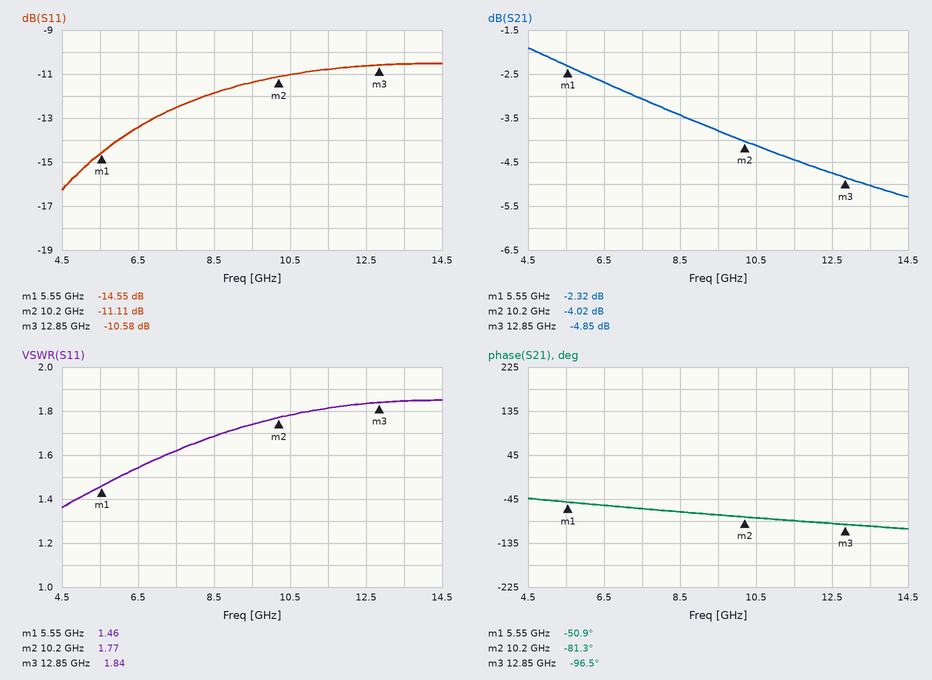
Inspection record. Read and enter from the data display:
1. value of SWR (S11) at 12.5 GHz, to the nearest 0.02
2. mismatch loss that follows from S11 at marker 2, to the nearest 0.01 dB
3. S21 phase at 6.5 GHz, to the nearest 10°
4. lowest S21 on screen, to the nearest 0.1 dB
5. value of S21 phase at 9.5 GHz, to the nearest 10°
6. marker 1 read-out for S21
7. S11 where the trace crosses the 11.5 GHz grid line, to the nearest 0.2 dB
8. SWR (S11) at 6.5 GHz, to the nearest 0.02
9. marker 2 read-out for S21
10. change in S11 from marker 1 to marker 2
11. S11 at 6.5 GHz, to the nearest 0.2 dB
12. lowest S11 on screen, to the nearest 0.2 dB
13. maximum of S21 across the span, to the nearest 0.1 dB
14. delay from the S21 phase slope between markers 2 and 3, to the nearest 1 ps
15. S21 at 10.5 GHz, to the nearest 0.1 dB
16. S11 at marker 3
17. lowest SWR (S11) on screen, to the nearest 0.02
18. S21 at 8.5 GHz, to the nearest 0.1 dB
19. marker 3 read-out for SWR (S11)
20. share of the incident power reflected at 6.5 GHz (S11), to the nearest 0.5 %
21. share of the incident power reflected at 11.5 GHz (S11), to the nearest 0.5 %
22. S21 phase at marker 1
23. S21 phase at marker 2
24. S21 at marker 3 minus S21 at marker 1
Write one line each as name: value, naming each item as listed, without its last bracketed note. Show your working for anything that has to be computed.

value of SWR (S11) at 12.5 GHz, to the nearest 0.02: 1.84
mismatch loss that follows from S11 at marker 2, to the nearest 0.01 dB: −10 log10(1 − 10^(-11.11/10)) ≈ 0.35 dB
S21 phase at 6.5 GHz, to the nearest 10°: -60°
lowest S21 on screen, to the nearest 0.1 dB: -5.3 dB
value of S21 phase at 9.5 GHz, to the nearest 10°: -80°
marker 1 read-out for S21: -2.32 dB
S11 where the trace crosses the 11.5 GHz grid line, to the nearest 0.2 dB: -10.8 dB
SWR (S11) at 6.5 GHz, to the nearest 0.02: 1.54
marker 2 read-out for S21: -4.02 dB
change in S11 from marker 1 to marker 2: -11.11 − (-14.55) = 3.44 dB
S11 at 6.5 GHz, to the nearest 0.2 dB: -13.4 dB
lowest S11 on screen, to the nearest 0.2 dB: -16.2 dB
maximum of S21 across the span, to the nearest 0.1 dB: -1.9 dB
delay from the S21 phase slope between markers 2 and 3, to the nearest 1 ps: −(-96.5° − (-81.3°))/(360° × 2.65 GHz) ≈ 16 ps
S21 at 10.5 GHz, to the nearest 0.1 dB: -4.1 dB
S11 at marker 3: -10.58 dB
lowest SWR (S11) on screen, to the nearest 0.02: 1.36
S21 at 8.5 GHz, to the nearest 0.1 dB: -3.4 dB
marker 3 read-out for SWR: 1.84
share of the incident power reflected at 6.5 GHz (S11), to the nearest 0.5 %: 10^(-13.4/10) ≈ 4.57 %, so 4.5 % to the nearest 0.5 %
share of the incident power reflected at 11.5 GHz (S11), to the nearest 0.5 %: 10^(-10.8/10) ≈ 8.32 %, so 8.5 % to the nearest 0.5 %
S21 phase at marker 1: -50.9°
S21 phase at marker 2: -81.3°
S21 at marker 3 minus S21 at marker 1: -4.85 − (-2.32) = -2.53 dB
